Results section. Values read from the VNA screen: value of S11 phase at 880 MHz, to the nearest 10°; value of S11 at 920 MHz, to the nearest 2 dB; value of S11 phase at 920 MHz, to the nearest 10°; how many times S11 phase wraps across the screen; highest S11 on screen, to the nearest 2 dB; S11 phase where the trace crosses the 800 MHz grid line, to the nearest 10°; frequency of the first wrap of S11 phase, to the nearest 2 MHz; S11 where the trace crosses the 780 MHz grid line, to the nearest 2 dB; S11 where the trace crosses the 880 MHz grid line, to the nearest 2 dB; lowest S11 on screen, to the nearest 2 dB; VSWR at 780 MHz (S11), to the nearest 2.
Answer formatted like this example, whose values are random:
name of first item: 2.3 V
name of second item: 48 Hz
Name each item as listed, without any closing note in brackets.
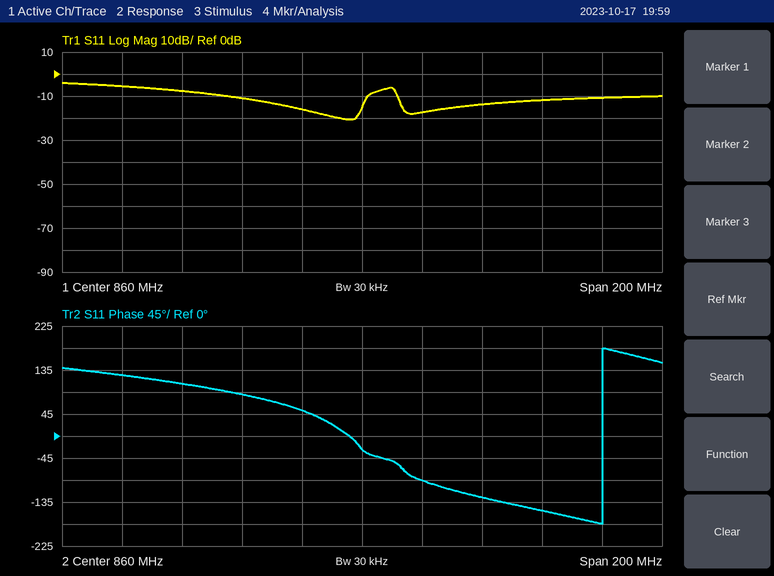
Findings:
value of S11 phase at 880 MHz, to the nearest 10°: -90°
value of S11 at 920 MHz, to the nearest 2 dB: -12 dB
value of S11 phase at 920 MHz, to the nearest 10°: -150°
how many times S11 phase wraps across the screen: 1
highest S11 on screen, to the nearest 2 dB: -4 dB
S11 phase where the trace crosses the 800 MHz grid line, to the nearest 10°: 110°
frequency of the first wrap of S11 phase, to the nearest 2 MHz: 940 MHz
S11 where the trace crosses the 780 MHz grid line, to the nearest 2 dB: -6 dB
S11 where the trace crosses the 880 MHz grid line, to the nearest 2 dB: -18 dB
lowest S11 on screen, to the nearest 2 dB: -20 dB
VSWR at 780 MHz (S11), to the nearest 2: 4
